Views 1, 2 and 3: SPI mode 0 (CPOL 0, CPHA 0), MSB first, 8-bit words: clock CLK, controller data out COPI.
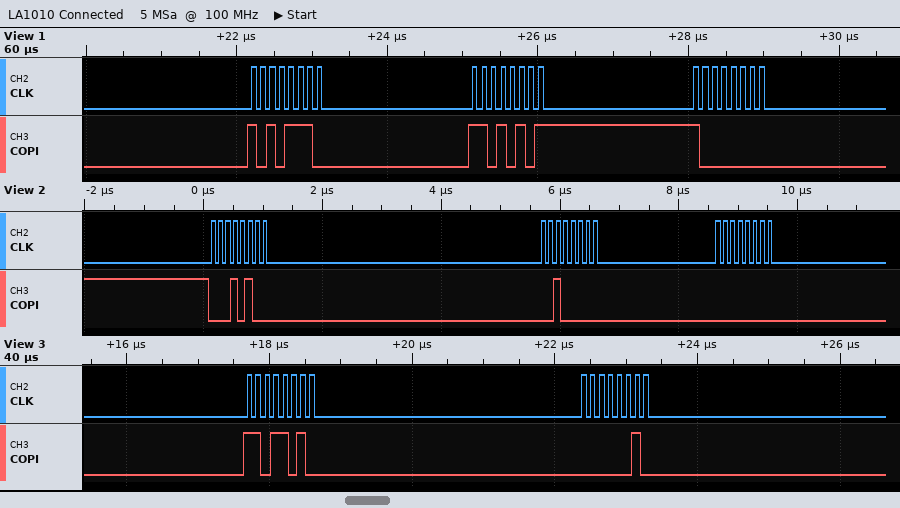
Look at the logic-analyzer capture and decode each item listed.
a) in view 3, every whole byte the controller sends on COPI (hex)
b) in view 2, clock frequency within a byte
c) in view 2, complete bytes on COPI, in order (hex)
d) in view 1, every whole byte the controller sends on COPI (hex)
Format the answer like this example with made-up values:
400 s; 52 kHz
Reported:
DA 02; 8 MHz; 14 20 00; AE D5 80
